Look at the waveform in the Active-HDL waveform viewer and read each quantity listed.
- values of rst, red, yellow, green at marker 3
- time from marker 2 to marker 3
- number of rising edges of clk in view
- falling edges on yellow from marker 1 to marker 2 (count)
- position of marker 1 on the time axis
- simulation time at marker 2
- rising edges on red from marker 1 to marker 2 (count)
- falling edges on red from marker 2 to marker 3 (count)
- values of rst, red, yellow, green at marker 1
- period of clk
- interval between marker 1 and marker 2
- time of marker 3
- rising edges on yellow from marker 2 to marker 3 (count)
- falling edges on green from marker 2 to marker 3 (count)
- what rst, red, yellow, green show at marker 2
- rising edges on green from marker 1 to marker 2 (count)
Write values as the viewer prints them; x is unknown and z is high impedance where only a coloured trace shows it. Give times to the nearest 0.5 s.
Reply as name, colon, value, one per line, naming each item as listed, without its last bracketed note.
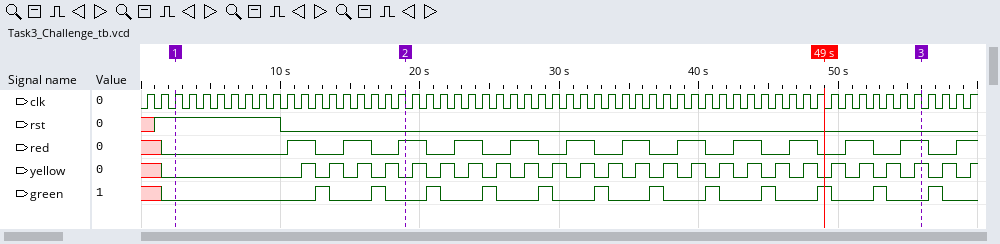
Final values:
values of rst, red, yellow, green at marker 3: rst=0, red=1, yellow=1, green=0
time from marker 2 to marker 3: 37 s
number of rising edges of clk in view: 60
falling edges on yellow from marker 1 to marker 2: 4
position of marker 1 on the time axis: 2.5 s
simulation time at marker 2: 19 s
rising edges on red from marker 1 to marker 2: 3
falling edges on red from marker 2 to marker 3: 9
values of rst, red, yellow, green at marker 1: rst=1, red=0, yellow=0, green=0
period of clk: 1 s
interval between marker 1 and marker 2: 16.5 s
time of marker 3: 56 s
rising edges on yellow from marker 2 to marker 3: 19
falling edges on green from marker 2 to marker 3: 9
what rst, red, yellow, green show at marker 2: rst=0, red=1, yellow=0, green=0
rising edges on green from marker 1 to marker 2: 2
